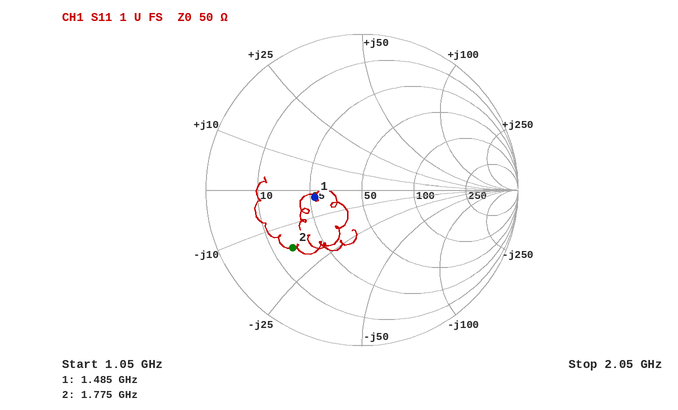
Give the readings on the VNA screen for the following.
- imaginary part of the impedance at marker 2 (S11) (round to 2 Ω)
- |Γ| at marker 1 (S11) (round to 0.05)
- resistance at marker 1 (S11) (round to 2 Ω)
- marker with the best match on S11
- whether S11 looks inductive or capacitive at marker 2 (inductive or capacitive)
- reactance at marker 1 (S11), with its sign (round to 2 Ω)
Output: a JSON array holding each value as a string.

["-16 Ω", "0.30", "26 Ω", "marker 1", "capacitive", "-2 Ω"]
